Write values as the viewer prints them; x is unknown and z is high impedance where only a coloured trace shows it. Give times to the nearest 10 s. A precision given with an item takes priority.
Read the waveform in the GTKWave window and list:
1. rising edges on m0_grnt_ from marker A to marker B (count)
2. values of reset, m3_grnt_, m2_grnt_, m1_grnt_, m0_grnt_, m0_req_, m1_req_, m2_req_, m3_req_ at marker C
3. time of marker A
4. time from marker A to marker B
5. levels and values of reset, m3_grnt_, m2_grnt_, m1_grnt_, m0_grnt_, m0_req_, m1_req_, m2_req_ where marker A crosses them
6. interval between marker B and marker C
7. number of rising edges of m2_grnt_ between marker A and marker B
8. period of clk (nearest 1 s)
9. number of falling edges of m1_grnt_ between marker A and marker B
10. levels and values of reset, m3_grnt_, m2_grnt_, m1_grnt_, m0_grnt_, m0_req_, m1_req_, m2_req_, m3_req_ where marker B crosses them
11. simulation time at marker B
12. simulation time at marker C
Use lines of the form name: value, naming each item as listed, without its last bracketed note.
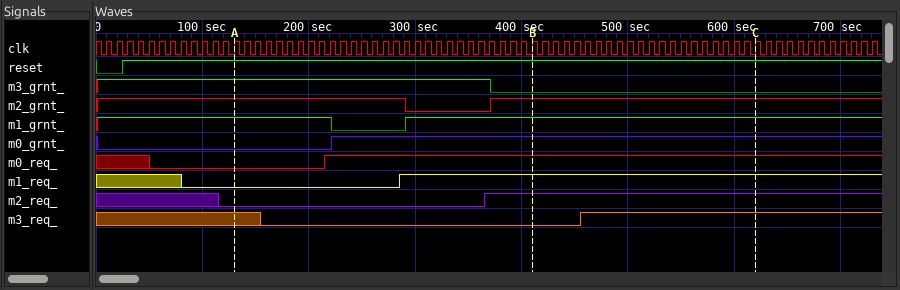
rising edges on m0_grnt_ from marker A to marker B: 1
values of reset, m3_grnt_, m2_grnt_, m1_grnt_, m0_grnt_, m0_req_, m1_req_, m2_req_, m3_req_ at marker C: reset=1, m3_grnt_=0, m2_grnt_=1, m1_grnt_=1, m0_grnt_=1, m0_req_=1, m1_req_=1, m2_req_=1, m3_req_=1
time of marker A: 130 s
time from marker A to marker B: 280 s
levels and values of reset, m3_grnt_, m2_grnt_, m1_grnt_, m0_grnt_, m0_req_, m1_req_, m2_req_ where marker A crosses them: reset=1, m3_grnt_=1, m2_grnt_=1, m1_grnt_=1, m0_grnt_=0, m0_req_=0, m1_req_=0, m2_req_=0
interval between marker B and marker C: 210 s
number of rising edges of m2_grnt_ between marker A and marker B: 1
period of clk: 10 s
number of falling edges of m1_grnt_ between marker A and marker B: 1
levels and values of reset, m3_grnt_, m2_grnt_, m1_grnt_, m0_grnt_, m0_req_, m1_req_, m2_req_, m3_req_ where marker B crosses them: reset=1, m3_grnt_=0, m2_grnt_=1, m1_grnt_=1, m0_grnt_=1, m0_req_=1, m1_req_=1, m2_req_=1, m3_req_=0
simulation time at marker B: 410 s
simulation time at marker C: 620 s
